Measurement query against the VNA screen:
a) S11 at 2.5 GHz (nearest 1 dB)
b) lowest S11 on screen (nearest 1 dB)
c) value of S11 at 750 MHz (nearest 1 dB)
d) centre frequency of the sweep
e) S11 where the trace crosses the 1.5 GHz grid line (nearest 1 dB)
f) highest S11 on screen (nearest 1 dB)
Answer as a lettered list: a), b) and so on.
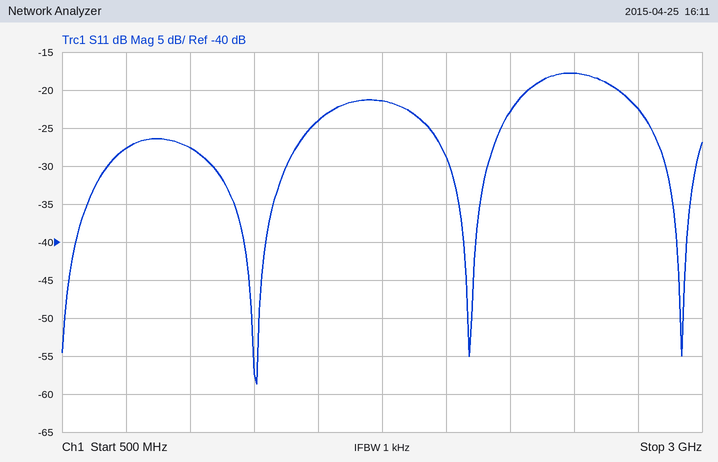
a) -18 dB
b) -59 dB
c) -28 dB
d) 1.75 GHz
e) -24 dB
f) -18 dB
